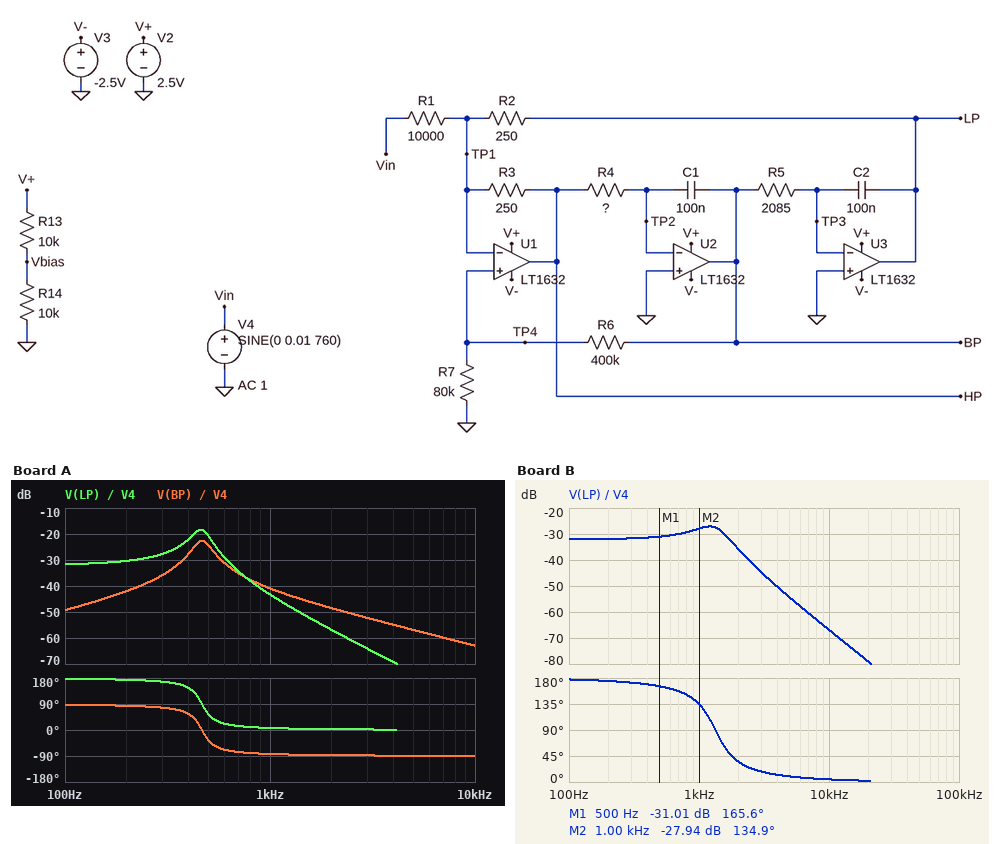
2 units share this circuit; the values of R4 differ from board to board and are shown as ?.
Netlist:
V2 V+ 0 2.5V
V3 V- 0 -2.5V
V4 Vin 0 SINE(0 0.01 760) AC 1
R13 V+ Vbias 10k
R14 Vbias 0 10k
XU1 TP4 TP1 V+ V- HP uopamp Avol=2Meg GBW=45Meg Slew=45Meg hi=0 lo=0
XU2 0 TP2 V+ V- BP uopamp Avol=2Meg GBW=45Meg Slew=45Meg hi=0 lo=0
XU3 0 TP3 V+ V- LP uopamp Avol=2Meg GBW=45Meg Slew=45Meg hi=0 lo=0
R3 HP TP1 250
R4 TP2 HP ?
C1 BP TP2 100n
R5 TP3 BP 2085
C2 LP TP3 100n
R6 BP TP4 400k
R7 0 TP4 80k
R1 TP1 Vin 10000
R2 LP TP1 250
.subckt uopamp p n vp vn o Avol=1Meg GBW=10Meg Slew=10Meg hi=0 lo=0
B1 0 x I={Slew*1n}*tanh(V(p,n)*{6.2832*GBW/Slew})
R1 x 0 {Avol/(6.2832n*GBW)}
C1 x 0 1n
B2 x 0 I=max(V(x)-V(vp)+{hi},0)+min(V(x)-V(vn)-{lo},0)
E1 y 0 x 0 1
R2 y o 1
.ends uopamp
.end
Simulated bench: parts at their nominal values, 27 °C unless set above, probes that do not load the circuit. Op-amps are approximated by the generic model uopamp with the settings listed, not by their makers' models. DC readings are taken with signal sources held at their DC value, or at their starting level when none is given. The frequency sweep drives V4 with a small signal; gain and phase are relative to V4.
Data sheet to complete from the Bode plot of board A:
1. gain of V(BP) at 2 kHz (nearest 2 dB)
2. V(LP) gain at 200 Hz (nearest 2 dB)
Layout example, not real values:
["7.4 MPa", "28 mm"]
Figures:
["-48 dB", "-30 dB"]
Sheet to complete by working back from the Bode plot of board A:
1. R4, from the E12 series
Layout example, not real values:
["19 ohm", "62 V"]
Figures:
["5.6 kΩ"]
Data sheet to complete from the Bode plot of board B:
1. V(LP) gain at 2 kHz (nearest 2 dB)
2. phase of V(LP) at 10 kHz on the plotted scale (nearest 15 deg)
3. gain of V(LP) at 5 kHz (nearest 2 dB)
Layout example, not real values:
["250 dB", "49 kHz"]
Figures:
["-36 dB", "0 deg", "-54 dB"]
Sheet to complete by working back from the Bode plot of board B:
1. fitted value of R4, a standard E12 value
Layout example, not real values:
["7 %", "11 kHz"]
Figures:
["680 Ω"]
